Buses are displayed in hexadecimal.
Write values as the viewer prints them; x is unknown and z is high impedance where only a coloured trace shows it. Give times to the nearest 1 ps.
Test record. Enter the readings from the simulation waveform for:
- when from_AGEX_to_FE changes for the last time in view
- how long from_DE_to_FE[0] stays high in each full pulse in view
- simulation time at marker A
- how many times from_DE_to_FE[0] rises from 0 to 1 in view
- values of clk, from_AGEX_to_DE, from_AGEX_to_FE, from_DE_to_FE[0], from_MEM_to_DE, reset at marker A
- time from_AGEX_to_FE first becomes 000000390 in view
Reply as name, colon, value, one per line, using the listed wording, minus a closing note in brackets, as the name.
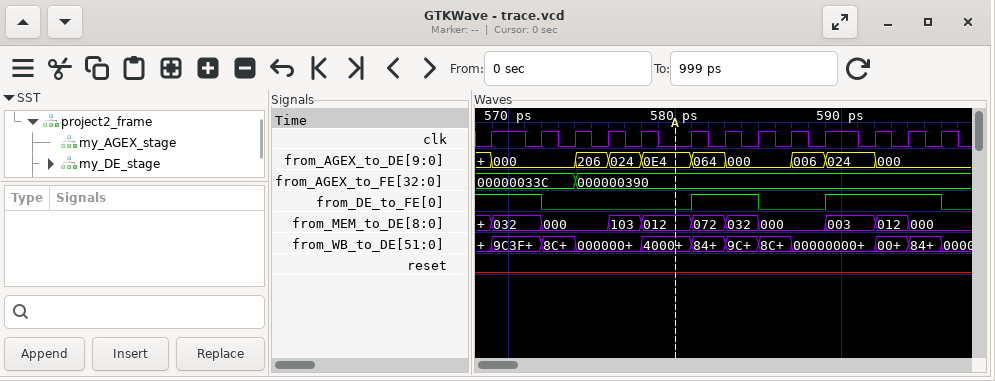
when from_AGEX_to_FE changes for the last time in view: 574 ps
how long from_DE_to_FE[0] stays high in each full pulse in view: 4 ps, 7 ps
simulation time at marker A: 580 ps
how many times from_DE_to_FE[0] rises from 0 to 1 in view: 2
values of clk, from_AGEX_to_DE, from_AGEX_to_FE, from_DE_to_FE[0], from_MEM_to_DE, reset at marker A: clk=0, from_AGEX_to_DE=0E4, from_AGEX_to_FE=000000390, from_DE_to_FE[0]=0, from_MEM_to_DE=012, reset=0
time from_AGEX_to_FE first becomes 000000390 in view: 574 ps
